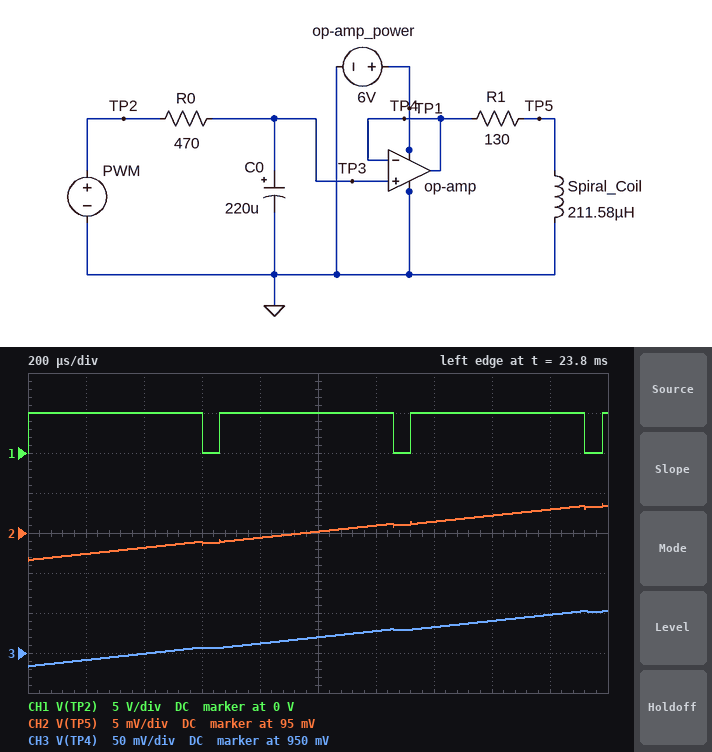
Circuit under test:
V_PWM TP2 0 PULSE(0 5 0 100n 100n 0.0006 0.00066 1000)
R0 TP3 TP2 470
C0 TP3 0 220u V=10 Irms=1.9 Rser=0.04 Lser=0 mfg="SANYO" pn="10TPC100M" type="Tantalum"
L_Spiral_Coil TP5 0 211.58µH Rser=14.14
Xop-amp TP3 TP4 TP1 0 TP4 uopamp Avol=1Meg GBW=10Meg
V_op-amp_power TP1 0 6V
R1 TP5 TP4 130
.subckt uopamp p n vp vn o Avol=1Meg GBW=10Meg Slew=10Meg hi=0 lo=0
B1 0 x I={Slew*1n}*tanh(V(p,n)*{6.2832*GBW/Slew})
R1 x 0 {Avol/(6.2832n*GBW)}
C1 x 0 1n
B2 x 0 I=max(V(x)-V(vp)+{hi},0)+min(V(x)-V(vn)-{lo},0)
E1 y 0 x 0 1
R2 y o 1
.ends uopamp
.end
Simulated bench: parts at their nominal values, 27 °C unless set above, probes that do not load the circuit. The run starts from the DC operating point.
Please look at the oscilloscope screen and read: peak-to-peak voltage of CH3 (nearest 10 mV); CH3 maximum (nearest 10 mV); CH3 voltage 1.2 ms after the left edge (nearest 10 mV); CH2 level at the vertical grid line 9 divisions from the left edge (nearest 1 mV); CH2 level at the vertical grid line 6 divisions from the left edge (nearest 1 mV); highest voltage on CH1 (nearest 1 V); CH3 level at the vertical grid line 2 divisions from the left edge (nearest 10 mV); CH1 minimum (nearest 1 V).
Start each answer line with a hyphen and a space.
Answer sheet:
- 70 mV
- 1.00 V
- 980 mV
- 98 mV
- 96 mV
- 5 V
- 950 mV
- 0 V
